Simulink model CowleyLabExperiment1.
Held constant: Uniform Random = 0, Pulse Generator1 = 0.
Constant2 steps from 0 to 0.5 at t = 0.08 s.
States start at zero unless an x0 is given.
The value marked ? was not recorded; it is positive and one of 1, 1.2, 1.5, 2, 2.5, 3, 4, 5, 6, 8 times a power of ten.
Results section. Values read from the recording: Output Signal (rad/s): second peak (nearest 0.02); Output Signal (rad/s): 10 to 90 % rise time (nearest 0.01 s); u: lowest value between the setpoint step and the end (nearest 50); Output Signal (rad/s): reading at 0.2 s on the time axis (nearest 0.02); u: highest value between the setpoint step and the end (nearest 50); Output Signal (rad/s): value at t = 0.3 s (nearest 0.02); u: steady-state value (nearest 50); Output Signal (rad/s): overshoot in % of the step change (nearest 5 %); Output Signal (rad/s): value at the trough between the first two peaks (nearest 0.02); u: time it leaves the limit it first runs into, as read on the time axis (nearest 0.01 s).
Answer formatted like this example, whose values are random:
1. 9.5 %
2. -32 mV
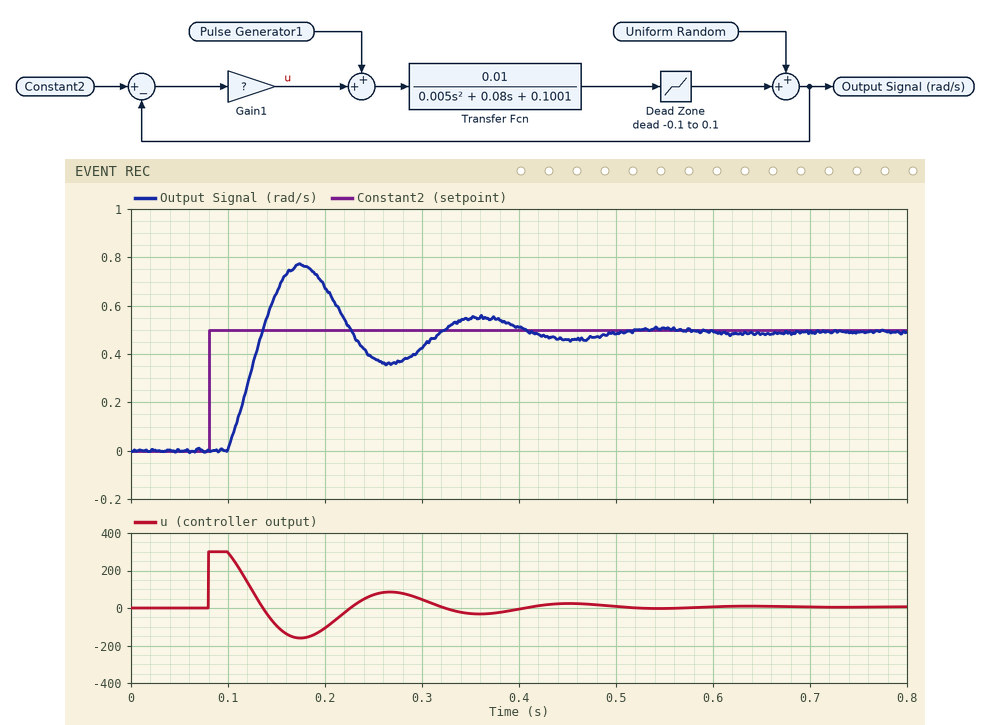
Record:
1. 0.56
2. 0.03 s
3. -150
4. 0.68
5. 300
6. 0.42
7. 0
8. 55 %
9. 0.36
10. 0.10 s
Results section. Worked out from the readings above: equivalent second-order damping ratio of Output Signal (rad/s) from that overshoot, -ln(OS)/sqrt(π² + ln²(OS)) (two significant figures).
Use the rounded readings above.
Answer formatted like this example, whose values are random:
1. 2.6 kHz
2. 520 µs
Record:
1. 0.19
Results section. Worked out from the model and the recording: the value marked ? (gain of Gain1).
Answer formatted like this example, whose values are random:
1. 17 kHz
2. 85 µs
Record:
1. 600
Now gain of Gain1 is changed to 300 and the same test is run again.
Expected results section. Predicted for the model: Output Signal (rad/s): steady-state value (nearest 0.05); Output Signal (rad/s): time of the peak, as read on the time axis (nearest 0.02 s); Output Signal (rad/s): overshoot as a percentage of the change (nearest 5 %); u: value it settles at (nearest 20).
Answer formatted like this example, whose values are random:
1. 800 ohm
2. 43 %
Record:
1. 0.50
2. 0.22 s
3. 40 %
4. 0
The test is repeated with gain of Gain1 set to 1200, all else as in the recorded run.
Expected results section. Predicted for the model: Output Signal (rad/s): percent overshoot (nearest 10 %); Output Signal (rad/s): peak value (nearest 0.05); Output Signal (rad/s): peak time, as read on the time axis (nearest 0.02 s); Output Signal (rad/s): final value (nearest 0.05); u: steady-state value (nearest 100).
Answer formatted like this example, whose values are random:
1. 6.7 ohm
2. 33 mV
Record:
1. 70 %
2. 0.85
3. 0.14 s
4. 0.50
5. 0
